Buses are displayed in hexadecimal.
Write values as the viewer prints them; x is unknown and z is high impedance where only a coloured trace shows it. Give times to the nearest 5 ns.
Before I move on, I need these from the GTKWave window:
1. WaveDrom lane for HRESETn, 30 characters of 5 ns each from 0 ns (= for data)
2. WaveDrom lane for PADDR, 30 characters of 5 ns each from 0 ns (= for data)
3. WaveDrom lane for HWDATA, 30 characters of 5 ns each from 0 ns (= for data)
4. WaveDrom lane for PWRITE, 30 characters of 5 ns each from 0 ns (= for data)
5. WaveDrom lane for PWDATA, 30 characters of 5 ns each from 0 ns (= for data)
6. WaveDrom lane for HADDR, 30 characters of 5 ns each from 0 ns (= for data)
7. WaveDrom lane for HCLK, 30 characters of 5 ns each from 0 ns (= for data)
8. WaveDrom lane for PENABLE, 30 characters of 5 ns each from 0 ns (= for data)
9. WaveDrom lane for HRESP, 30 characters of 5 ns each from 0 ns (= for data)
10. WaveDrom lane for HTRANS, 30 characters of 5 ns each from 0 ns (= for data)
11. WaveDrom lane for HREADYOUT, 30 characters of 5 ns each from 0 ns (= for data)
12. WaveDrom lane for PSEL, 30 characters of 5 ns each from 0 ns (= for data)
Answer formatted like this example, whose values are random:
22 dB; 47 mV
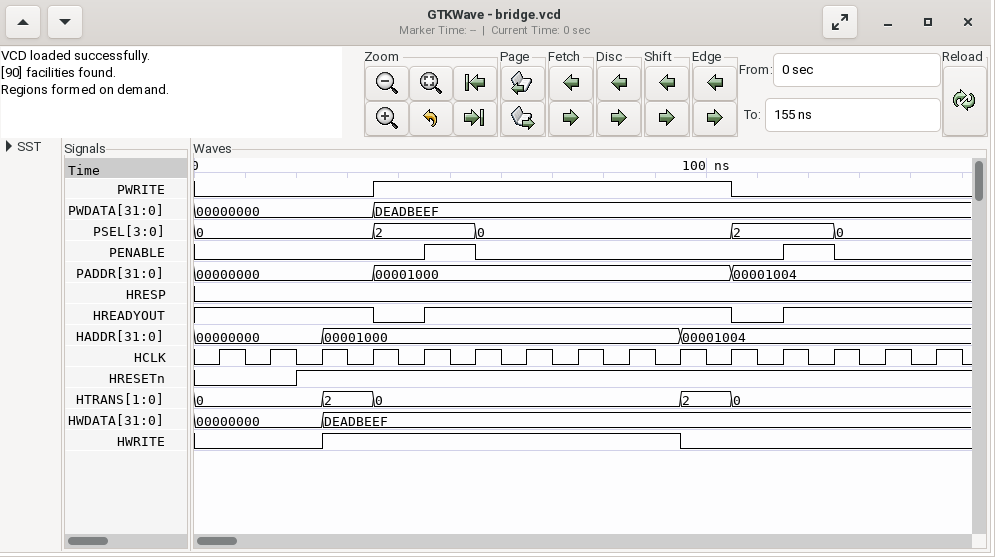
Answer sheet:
{name: 'HRESETn', wave: '0...1.........................'}; {name: 'PADDR', wave: '=......=.............=........', data: '00000000 00001000 00001004'}; {name: 'HWDATA', wave: '=....=........................', data: '00000000 DEADBEEF'}; {name: 'PWRITE', wave: '0......1.............0........'}; {name: 'PWDATA', wave: '=......=......................', data: '00000000 DEADBEEF'}; {name: 'HADDR', wave: '=....=.............=..........', data: '00000000 00001000 00001004'}; {name: 'HCLK', wave: '010101010101010101010101010101'}; {name: 'PENABLE', wave: '0........1.0...........1.0....'}; {name: 'HRESP', wave: '0.............................'}; {name: 'HTRANS', wave: '=....=.=...........=.=........', data: '0 2 0 2 0'}; {name: 'HREADYOUT', wave: '1......0.1...........0.1......'}; {name: 'PSEL', wave: '=......=...=.........=...=....', data: '0 2 0 2 0'}
